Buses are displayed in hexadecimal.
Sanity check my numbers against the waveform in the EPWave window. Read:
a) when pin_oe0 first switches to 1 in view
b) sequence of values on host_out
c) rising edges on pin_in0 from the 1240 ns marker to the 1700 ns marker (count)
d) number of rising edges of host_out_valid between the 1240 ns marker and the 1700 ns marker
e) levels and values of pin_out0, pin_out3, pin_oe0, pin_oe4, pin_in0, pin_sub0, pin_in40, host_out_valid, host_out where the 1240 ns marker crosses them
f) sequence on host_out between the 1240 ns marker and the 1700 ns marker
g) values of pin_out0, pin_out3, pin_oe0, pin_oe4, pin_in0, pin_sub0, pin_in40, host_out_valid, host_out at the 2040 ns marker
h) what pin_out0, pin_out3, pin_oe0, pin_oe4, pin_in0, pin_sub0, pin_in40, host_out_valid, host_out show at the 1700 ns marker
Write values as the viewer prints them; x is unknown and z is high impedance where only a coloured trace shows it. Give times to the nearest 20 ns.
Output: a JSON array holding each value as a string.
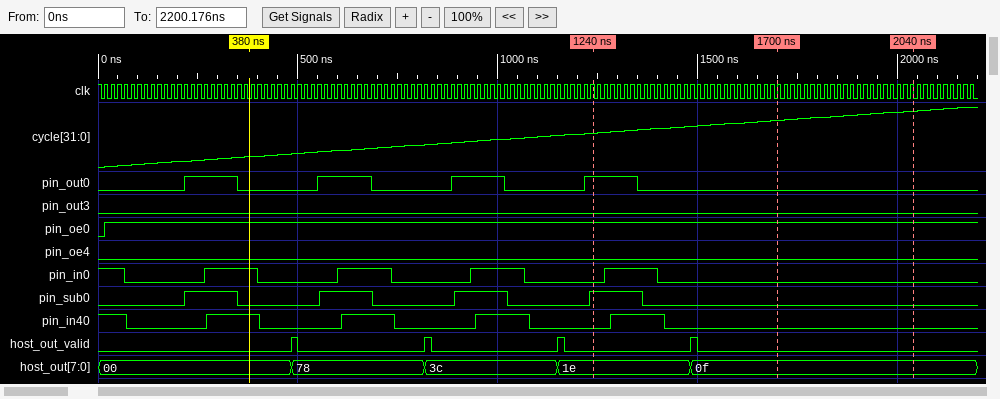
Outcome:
["20 ns", "00, 78, 3c, 1e, 0f", "1", "1", "pin_out0=1, pin_out3=0, pin_oe0=1, pin_oe4=0, pin_in0=0, pin_sub0=1, pin_in40=0, host_out_valid=0, host_out=1e", "1e, 0f", "pin_out0=0, pin_out3=0, pin_oe0=1, pin_oe4=0, pin_in0=0, pin_sub0=0, pin_in40=0, host_out_valid=0, host_out=0f", "pin_out0=0, pin_out3=0, pin_oe0=1, pin_oe4=0, pin_in0=0, pin_sub0=0, pin_in40=0, host_out_valid=0, host_out=0f"]
